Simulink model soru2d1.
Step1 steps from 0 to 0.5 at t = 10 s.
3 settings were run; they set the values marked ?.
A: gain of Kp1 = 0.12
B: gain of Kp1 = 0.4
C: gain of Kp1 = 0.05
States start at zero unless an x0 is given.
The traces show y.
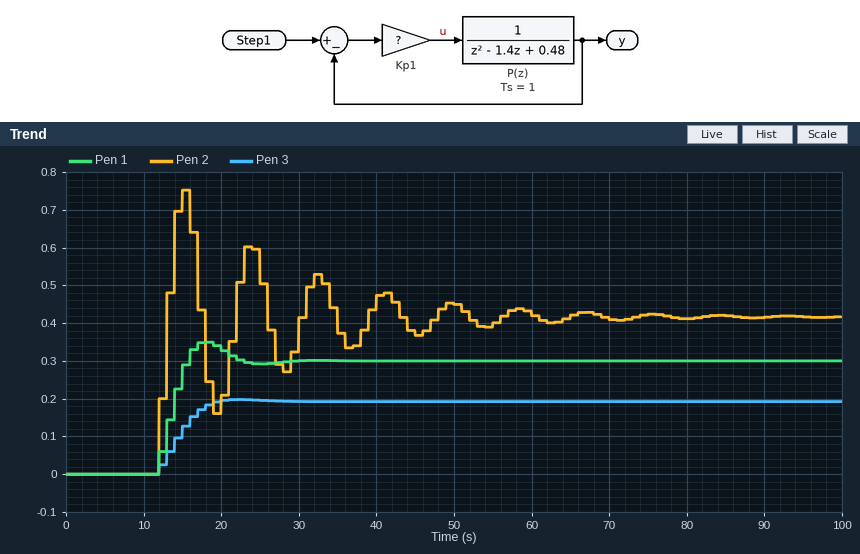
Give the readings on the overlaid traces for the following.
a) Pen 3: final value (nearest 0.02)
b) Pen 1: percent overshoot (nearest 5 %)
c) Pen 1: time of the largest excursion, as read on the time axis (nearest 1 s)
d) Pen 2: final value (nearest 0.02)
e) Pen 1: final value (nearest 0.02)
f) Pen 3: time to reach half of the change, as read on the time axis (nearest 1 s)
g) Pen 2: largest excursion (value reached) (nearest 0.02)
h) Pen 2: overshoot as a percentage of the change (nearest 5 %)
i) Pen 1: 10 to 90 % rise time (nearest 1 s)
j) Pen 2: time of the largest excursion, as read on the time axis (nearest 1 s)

0.20
15 %
18 s
0.42
0.30
15 s
0.76
80 %
3 s
15 s
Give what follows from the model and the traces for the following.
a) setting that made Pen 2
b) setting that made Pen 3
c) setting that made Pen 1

B
C
A
